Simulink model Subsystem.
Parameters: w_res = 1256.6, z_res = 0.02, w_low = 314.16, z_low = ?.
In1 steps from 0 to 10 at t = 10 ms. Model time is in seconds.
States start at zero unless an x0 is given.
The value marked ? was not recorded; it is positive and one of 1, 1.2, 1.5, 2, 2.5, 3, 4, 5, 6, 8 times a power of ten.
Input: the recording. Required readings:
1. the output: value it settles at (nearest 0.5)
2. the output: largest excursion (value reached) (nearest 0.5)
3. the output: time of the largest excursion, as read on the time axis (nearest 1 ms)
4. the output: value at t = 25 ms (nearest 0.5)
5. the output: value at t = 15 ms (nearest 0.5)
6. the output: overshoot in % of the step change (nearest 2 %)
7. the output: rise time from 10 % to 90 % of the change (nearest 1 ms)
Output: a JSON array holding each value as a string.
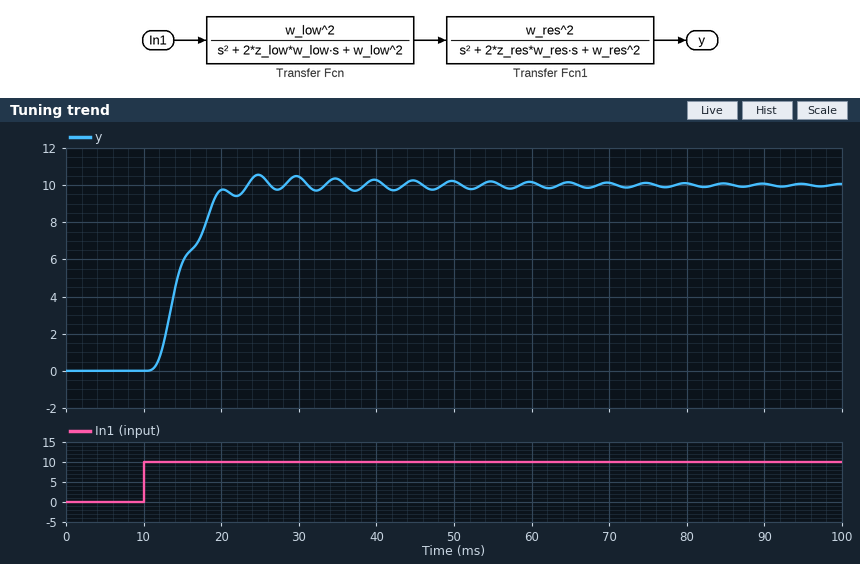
["10.0", "10.5", "25 ms", "10.5", "6.0", "6 %", "7 ms"]
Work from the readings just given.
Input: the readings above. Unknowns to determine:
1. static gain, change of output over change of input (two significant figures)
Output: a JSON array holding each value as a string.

["1.0"]
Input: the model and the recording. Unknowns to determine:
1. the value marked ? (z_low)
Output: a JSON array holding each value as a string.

["0.8"]
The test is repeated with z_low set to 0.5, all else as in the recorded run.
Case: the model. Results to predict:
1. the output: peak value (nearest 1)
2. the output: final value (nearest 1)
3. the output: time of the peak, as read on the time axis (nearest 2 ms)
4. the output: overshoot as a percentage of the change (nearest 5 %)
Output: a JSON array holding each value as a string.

["12", "10", "20 ms", "20 %"]
